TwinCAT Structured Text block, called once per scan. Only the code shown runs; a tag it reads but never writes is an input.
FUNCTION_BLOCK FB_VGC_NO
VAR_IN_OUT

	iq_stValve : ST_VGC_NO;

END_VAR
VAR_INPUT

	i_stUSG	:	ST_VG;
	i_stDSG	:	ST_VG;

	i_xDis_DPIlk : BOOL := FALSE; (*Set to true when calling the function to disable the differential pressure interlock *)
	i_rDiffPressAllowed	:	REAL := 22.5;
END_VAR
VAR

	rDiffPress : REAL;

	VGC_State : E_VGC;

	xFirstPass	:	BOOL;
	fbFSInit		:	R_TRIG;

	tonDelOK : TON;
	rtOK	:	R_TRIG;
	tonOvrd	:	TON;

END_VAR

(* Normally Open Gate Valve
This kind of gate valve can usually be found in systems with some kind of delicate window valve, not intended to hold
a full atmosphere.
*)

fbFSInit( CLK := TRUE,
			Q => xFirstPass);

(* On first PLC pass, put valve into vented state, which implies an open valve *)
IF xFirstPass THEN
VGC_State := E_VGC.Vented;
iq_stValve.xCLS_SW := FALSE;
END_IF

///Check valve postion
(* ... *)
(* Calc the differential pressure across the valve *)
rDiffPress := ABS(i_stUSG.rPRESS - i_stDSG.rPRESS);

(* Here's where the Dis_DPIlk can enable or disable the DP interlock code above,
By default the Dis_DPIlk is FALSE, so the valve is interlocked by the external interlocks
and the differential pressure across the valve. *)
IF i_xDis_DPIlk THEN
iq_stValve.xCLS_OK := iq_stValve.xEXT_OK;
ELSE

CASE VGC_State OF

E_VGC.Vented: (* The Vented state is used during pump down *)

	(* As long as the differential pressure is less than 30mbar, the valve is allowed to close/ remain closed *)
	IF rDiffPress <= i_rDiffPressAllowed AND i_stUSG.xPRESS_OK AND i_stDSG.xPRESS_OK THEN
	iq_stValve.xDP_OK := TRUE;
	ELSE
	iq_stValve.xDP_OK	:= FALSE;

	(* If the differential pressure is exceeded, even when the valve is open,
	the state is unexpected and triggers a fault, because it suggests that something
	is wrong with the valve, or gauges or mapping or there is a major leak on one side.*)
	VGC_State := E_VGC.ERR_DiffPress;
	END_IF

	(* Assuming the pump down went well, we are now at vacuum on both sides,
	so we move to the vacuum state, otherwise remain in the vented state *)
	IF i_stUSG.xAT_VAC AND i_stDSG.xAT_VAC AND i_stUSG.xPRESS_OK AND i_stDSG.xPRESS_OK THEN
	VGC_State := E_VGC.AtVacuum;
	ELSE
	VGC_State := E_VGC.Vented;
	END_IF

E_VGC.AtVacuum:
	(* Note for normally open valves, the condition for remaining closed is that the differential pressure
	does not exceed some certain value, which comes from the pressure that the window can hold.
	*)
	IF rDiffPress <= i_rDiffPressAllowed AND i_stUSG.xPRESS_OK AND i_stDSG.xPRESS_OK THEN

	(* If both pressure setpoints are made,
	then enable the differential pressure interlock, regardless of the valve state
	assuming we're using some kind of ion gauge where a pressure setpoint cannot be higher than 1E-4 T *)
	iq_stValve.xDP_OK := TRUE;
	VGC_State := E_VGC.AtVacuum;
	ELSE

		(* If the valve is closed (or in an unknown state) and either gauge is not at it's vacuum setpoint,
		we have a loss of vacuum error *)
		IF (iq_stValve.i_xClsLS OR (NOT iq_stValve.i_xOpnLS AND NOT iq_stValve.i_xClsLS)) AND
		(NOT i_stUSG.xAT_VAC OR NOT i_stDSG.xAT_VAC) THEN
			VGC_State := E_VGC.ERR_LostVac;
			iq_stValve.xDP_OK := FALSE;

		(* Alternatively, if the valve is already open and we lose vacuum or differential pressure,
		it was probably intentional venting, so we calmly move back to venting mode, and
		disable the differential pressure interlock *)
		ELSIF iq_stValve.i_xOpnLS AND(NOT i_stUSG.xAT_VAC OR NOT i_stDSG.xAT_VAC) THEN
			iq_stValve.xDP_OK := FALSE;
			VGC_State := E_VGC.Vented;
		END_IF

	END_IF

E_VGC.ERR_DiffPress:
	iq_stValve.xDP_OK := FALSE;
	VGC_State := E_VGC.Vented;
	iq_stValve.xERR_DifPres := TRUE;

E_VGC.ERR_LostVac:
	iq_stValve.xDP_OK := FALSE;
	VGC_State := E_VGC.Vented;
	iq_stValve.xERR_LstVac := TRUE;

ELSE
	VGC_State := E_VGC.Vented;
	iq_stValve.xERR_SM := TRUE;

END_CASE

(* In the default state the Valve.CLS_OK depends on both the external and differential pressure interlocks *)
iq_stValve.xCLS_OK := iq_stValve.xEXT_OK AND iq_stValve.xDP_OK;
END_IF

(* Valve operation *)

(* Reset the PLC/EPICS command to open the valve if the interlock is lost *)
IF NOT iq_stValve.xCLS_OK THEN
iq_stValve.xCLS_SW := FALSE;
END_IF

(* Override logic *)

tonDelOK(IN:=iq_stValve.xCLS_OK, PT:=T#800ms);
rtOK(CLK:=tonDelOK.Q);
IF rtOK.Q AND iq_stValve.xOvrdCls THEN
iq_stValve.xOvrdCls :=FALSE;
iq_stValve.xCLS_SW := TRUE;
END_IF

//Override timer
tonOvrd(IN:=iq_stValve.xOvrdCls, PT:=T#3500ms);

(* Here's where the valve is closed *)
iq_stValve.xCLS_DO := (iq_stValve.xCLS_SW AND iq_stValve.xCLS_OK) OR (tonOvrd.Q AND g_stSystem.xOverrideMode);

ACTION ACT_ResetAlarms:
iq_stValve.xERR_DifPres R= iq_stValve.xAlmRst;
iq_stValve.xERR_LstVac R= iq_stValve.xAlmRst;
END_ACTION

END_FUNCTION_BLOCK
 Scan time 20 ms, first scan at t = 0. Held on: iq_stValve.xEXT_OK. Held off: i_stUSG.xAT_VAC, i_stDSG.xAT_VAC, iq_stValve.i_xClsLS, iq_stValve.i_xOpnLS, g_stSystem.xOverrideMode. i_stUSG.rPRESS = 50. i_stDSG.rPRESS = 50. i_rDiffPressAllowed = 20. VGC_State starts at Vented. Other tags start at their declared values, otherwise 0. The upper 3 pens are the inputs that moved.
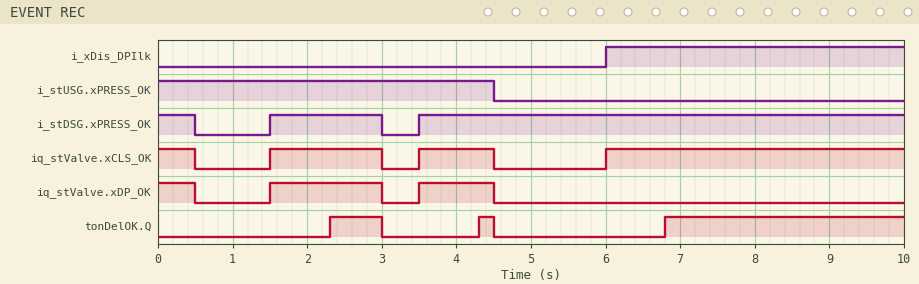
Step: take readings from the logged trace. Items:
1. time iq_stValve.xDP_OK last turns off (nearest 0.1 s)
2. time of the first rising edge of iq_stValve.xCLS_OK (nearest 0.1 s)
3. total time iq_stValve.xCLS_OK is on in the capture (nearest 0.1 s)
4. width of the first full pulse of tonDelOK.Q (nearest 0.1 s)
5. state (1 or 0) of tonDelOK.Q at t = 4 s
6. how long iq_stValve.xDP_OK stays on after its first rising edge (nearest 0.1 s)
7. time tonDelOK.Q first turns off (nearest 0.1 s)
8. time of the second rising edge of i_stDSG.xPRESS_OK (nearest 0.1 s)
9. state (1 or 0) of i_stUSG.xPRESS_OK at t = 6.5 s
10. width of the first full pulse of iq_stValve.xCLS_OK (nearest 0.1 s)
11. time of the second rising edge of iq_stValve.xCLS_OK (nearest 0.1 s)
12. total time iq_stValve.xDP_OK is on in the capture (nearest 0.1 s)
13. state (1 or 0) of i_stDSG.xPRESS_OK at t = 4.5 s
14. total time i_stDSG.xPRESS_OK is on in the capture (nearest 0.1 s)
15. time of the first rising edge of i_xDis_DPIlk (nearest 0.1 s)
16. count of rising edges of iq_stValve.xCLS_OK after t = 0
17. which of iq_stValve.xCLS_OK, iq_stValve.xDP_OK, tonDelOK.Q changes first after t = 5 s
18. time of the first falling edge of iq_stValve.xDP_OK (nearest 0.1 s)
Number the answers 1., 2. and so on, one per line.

1. 4.5 s
2. 1.5 s
3. 7.0 s
4. 0.7 s
5. 0
6. 1.5 s
7. 3.0 s
8. 3.5 s
9. 0
10. 1.5 s
11. 3.5 s
12. 3.0 s
13. 1
14. 8.5 s
15. 6.0 s
16. 3
17. iq_stValve.xCLS_OK
18. 0.5 s
